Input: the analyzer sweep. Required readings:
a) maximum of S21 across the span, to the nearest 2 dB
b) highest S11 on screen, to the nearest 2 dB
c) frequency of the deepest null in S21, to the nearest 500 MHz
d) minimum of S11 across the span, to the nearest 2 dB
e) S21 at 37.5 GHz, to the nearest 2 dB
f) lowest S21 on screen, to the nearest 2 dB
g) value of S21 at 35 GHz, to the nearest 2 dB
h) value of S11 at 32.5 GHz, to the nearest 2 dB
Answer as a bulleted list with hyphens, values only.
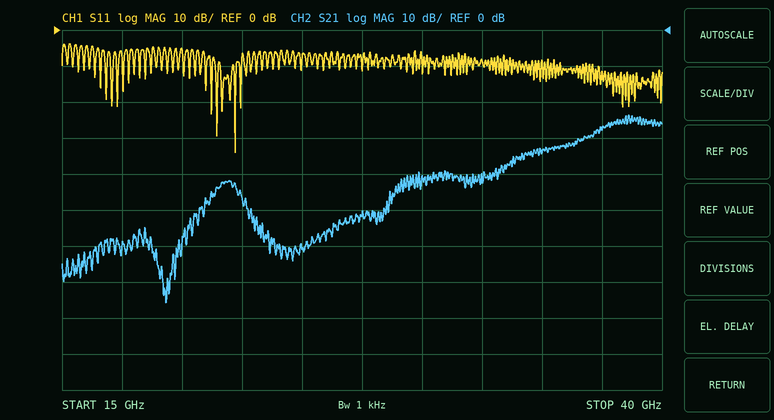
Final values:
- -24 dB
- -4 dB
- 19.5 GHz
- -34 dB
- -28 dB
- -76 dB
- -34 dB
- -8 dB
